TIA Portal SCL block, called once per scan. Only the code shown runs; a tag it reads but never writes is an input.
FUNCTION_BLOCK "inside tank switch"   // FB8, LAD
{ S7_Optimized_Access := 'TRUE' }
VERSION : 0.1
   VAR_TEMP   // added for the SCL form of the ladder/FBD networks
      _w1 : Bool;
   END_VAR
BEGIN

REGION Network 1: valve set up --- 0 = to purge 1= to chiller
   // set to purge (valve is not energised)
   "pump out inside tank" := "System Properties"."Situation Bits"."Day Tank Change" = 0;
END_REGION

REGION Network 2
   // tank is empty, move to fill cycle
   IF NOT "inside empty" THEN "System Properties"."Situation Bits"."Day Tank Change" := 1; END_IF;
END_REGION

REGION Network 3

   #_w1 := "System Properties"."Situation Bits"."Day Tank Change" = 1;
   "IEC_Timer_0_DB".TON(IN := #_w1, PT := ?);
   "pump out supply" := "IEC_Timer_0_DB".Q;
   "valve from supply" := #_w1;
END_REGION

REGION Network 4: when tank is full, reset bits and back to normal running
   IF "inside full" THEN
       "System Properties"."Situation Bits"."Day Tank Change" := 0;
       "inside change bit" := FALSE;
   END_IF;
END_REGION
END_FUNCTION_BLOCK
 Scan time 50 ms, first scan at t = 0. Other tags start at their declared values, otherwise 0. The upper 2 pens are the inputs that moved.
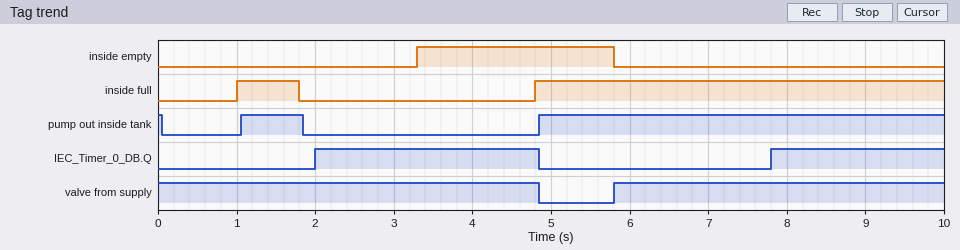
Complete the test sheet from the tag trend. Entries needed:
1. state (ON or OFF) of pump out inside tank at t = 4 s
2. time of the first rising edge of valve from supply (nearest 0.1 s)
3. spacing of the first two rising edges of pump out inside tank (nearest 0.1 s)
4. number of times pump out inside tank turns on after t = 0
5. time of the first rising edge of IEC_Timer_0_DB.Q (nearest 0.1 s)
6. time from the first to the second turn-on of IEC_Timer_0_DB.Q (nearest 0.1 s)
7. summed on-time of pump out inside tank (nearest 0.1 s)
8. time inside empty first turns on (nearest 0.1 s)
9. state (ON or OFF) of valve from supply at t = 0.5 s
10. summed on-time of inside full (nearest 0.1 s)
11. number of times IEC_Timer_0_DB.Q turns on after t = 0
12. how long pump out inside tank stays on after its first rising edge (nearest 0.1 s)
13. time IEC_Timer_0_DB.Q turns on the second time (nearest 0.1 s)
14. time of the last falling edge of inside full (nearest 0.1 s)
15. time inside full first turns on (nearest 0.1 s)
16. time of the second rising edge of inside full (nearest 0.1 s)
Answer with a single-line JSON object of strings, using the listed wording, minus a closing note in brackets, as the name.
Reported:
{"state (ON or OFF) of pump out inside tank at t = 4 s": "OFF", "time of the first rising edge of valve from supply": "5.8 s", "spacing of the first two rising edges of pump out inside tank": "3.8 s", "number of times pump out inside tank turns on after t = 0": "2", "time of the first rising edge of IEC_Timer_0_DB.Q": "2.0 s", "time from the first to the second turn-on of IEC_Timer_0_DB.Q": "5.8 s", "summed on-time of pump out inside tank": "6.0 s", "time inside empty first turns on": "3.3 s", "state (ON or OFF) of valve from supply at t = 0.5 s": "ON", "summed on-time of inside full": "6.0 s", "number of times IEC_Timer_0_DB.Q turns on after t = 0": "2", "how long pump out inside tank stays on after its first rising edge": "0.8 s", "time IEC_Timer_0_DB.Q turns on the second time": "7.8 s", "time of the last falling edge of inside full": "1.8 s", "time inside full first turns on": "1.0 s", "time of the second rising edge of inside full": "4.8 s"}
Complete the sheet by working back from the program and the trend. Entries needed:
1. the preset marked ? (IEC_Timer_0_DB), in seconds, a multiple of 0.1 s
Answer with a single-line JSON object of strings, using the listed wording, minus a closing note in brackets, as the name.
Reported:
{"the preset marked ? (IEC_Timer_0_DB), in seconds, a multiple of 0.1 s": "2.0 s"}
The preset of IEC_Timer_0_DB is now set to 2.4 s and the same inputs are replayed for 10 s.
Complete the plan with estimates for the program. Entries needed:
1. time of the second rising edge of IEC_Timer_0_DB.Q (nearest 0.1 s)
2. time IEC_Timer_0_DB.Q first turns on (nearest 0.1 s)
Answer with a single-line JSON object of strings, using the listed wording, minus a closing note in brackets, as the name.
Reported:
{"time of the second rising edge of IEC_Timer_0_DB.Q": "8.2 s", "time IEC_Timer_0_DB.Q first turns on": "2.4 s"}
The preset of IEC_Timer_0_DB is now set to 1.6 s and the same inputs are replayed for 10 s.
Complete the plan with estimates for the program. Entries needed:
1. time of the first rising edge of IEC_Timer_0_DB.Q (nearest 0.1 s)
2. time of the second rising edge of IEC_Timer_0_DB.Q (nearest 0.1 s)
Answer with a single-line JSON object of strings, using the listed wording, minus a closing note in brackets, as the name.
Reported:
{"time of the first rising edge of IEC_Timer_0_DB.Q": "1.6 s", "time of the second rising edge of IEC_Timer_0_DB.Q": "7.4 s"}
